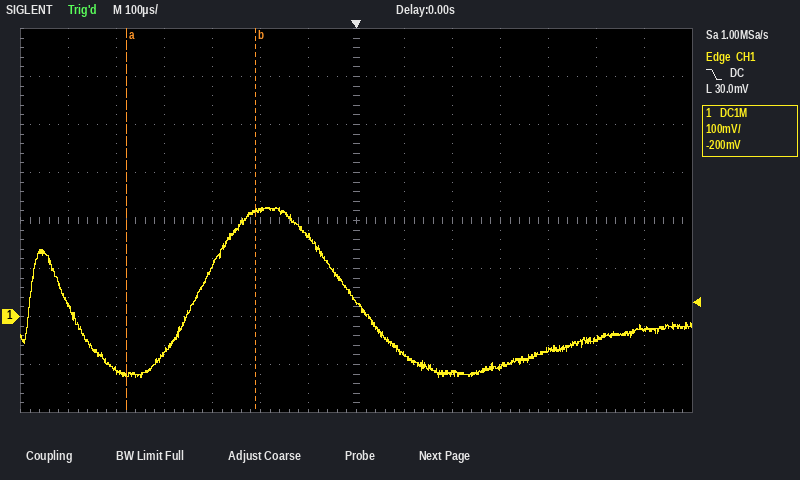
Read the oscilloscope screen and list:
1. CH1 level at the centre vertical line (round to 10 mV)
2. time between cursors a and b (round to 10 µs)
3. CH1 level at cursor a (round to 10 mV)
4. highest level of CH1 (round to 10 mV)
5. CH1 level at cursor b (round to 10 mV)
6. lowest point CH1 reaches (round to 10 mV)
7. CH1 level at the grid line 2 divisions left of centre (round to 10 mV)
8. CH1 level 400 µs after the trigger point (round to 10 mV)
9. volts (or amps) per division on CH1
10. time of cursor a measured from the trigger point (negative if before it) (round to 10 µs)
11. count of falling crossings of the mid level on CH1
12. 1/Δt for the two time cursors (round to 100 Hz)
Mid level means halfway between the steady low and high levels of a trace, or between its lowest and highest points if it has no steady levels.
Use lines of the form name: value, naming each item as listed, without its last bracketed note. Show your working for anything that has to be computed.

CH1 level at the centre vertical line: 30 mV
time between cursors a and b: 270 µs
CH1 level at cursor a: -120 mV
highest level of CH1: 230 mV
CH1 level at cursor b: 220 mV
lowest point CH1 reaches: -130 mV
CH1 level at the grid line 2 divisions left of centre: 220 mV
CH1 level 400 µs after the trigger point: -70 mV
volts (or amps) per division on CH1: 100 mV
time of cursor a measured from the trigger point (negative if before it): -480 µs
count of falling crossings of the mid level on CH1: 2
1/Δt for the two time cursors: 1 / 270 µs ≈ 3.7 kHz
